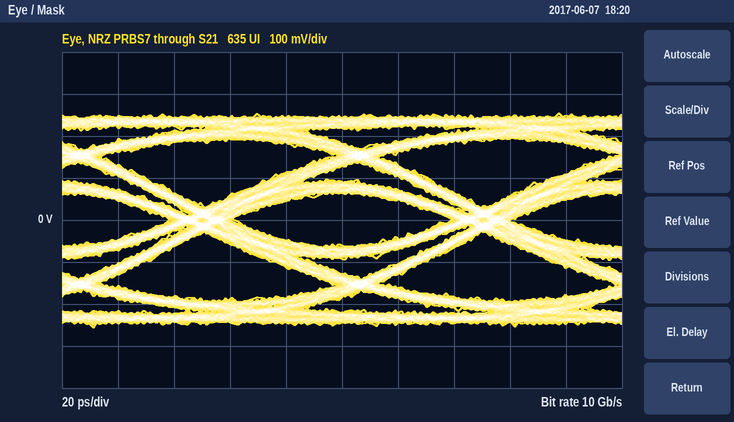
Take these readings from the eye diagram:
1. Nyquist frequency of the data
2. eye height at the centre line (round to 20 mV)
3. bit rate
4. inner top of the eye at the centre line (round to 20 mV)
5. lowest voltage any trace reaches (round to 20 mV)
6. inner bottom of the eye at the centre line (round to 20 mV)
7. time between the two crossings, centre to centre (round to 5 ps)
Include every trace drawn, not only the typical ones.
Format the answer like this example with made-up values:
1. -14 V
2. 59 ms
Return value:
1. 5 GHz
2. 120 mV
3. 10 Gb/s
4. 60 mV
5. -260 mV
6. -60 mV
7. 100 ps
